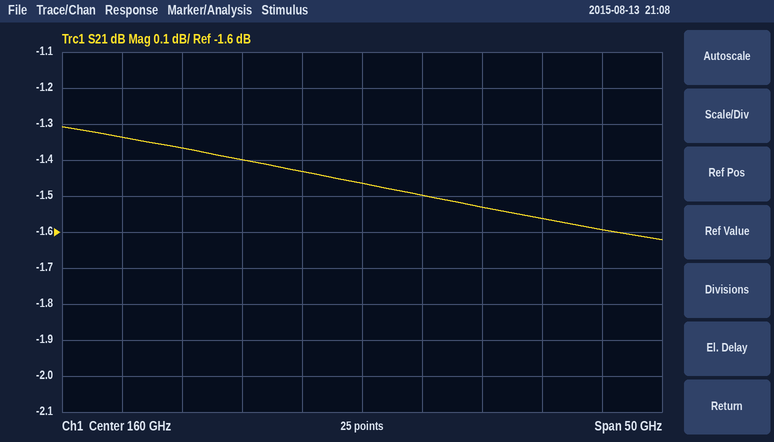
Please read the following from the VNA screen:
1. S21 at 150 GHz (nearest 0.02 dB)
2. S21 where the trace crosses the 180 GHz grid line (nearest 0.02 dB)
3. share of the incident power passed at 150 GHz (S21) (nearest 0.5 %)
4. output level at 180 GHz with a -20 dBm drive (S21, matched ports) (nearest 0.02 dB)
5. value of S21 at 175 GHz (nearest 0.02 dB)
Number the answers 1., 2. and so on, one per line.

1. -1.40 dB
2. -1.60 dB
3. 72.5 %
4. -21.60 dBm
5. -1.56 dB
